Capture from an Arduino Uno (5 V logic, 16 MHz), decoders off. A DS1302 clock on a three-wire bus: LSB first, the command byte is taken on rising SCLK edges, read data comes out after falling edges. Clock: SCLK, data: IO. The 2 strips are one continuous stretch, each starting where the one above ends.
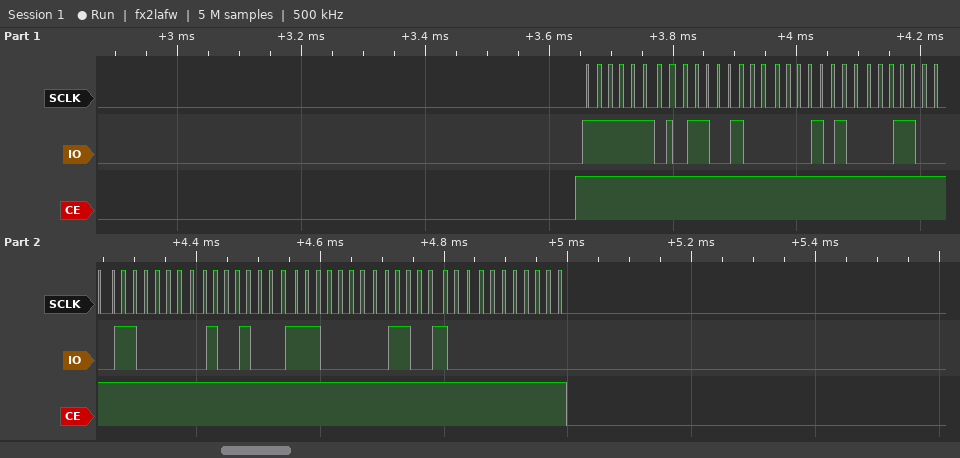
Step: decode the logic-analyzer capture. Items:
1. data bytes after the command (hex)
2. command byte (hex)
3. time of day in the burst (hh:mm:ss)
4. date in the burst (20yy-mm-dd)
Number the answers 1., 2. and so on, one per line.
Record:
1. 26 50 18 06 12 07 26 00
2. 0xBF
3. 18:50:26
4. 2026-12-06
